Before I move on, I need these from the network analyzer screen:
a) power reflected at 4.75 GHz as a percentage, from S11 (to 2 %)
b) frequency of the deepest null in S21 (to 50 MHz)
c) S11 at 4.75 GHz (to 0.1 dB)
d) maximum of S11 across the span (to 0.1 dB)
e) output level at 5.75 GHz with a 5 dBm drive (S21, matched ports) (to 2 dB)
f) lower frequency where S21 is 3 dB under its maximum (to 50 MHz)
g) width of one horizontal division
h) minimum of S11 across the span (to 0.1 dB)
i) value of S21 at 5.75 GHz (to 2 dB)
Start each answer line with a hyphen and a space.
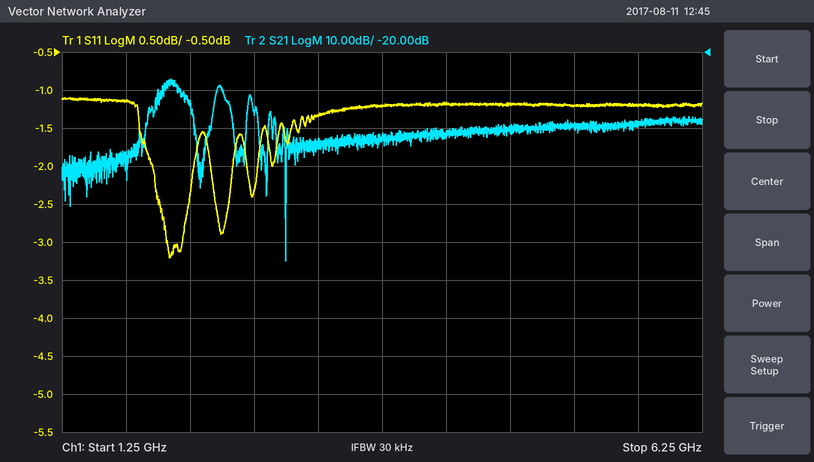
- 76 %
- 3.00 GHz
- -1.2 dB
- -1.1 dB
- -34 dBm
- 2.05 GHz
- 500 MHz
- -3.2 dB
- -38 dB
